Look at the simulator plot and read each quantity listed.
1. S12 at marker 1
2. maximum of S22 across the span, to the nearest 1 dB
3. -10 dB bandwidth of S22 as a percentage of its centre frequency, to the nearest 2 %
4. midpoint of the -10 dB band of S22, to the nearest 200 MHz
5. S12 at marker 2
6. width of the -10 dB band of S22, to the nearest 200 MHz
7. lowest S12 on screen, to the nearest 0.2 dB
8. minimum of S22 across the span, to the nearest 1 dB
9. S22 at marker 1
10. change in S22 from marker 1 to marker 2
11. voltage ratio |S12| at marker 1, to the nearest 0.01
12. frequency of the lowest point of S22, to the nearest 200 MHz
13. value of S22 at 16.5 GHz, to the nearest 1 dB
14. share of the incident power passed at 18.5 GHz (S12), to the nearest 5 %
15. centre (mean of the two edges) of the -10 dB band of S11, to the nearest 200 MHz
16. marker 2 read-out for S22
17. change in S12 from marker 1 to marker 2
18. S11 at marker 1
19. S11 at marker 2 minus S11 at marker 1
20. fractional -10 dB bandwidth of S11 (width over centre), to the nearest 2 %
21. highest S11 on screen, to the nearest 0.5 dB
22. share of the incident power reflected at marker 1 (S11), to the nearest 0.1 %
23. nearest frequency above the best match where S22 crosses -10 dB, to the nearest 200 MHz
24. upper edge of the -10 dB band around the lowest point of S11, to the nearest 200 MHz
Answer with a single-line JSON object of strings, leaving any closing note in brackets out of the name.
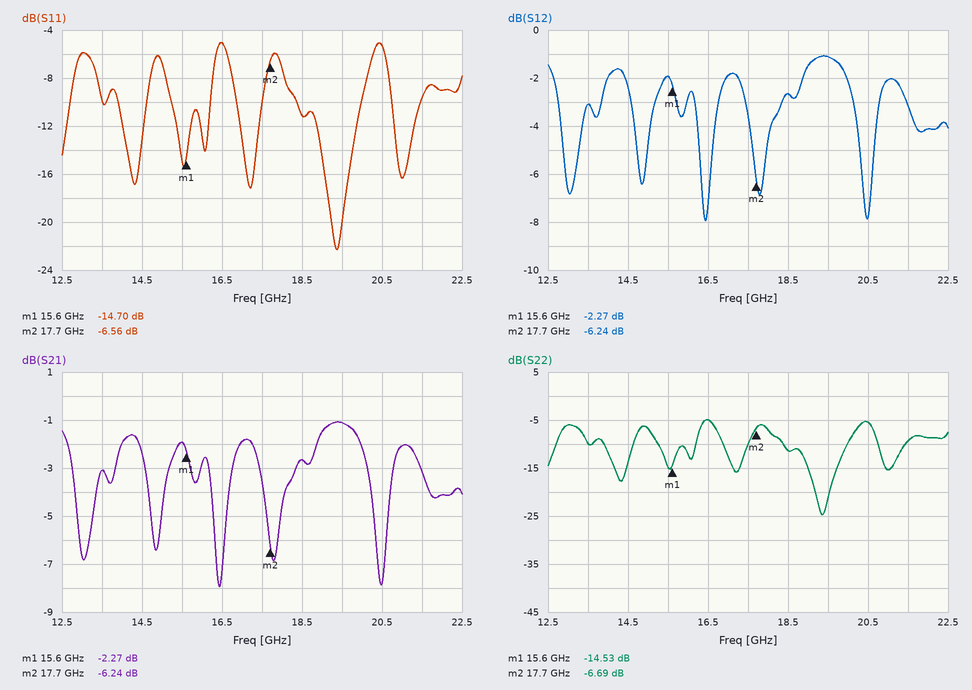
{"S12 at marker 1": "-2.27 dB", "maximum of S22 across the span, to the nearest 1 dB": "-5 dB", "-10 dB bandwidth of S22 as a percentage of its centre frequency, to the nearest 2 %": "8 %", "midpoint of the -10 dB band of S22, to the nearest 200 MHz": "19.2 GHz", "S12 at marker 2": "-6.24 dB", "width of the -10 dB band of S22, to the nearest 200 MHz": "1.6 GHz", "lowest S12 on screen, to the nearest 0.2 dB": "-8.0 dB", "minimum of S22 across the span, to the nearest 1 dB": "-25 dB", "S22 at marker 1": "-14.53 dB", "change in S22 from marker 1 to marker 2": "7.84 dB", "voltage ratio |S12| at marker 1, to the nearest 0.01": "0.77", "frequency of the lowest point of S22, to the nearest 200 MHz": "19.4 GHz", "value of S22 at 16.5 GHz, to the nearest 1 dB": "-5 dB", "share of the incident power passed at 18.5 GHz (S12), to the nearest 5 %": "55 %", "centre (mean of the two edges) of the -10 dB band of S11, to the nearest 200 MHz": "19.2 GHz", "marker 2 read-out for S22": "-6.69 dB", "change in S12 from marker 1 to marker 2": "-3.97 dB", "S11 at marker 1": "-14.70 dB", "S11 at marker 2 minus S11 at marker 1": "8.14 dB", "fractional -10 dB bandwidth of S11 (width over centre), to the nearest 2 %": "8 %", "highest S11 on screen, to the nearest 0.5 dB": "-5.0 dB", "share of the incident power reflected at marker 1 (S11), to the nearest 0.1 %": "3.4 %", "nearest frequency above the best match where S22 crosses -10 dB, to the nearest 200 MHz": "20.0 GHz", "upper edge of the -10 dB band around the lowest point of S11, to the nearest 200 MHz": "20.0 GHz"}
